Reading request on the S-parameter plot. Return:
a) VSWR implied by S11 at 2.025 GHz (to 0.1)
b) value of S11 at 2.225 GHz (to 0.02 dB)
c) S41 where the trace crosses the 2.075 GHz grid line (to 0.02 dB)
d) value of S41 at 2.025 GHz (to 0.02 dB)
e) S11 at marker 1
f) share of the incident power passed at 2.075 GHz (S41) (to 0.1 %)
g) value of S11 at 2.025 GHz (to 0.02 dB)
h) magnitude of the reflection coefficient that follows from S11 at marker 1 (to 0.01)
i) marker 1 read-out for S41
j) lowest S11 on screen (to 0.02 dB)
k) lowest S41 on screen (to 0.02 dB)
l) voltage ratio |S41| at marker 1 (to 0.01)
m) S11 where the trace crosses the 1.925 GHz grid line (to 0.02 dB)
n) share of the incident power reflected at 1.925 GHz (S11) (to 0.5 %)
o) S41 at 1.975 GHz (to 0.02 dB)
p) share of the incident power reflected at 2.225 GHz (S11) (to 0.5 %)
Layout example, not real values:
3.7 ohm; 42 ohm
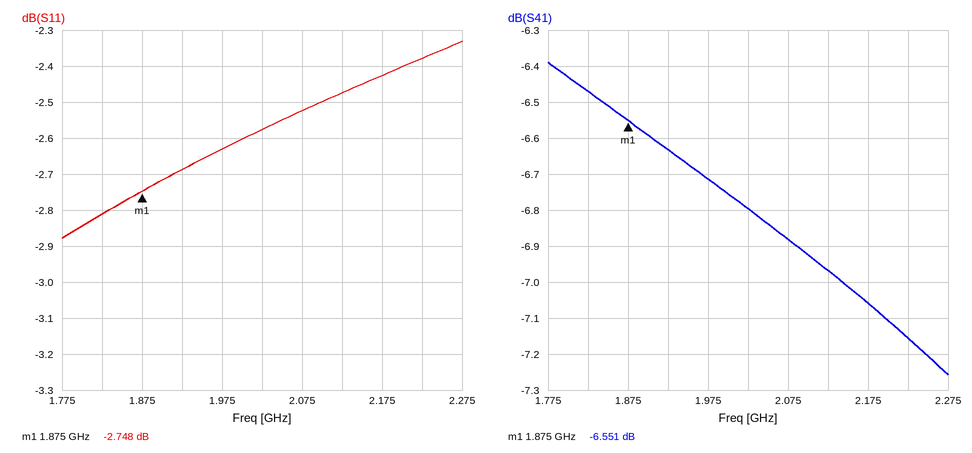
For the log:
6.8; -2.38 dB; -6.88 dB; -6.80 dB; -2.748 dB; 20.5 %; -2.58 dB; 0.73; -6.551 dB; -2.88 dB; -7.26 dB; 0.47; -2.68 dB; 54.0 %; -6.72 dB; 58.0 %
